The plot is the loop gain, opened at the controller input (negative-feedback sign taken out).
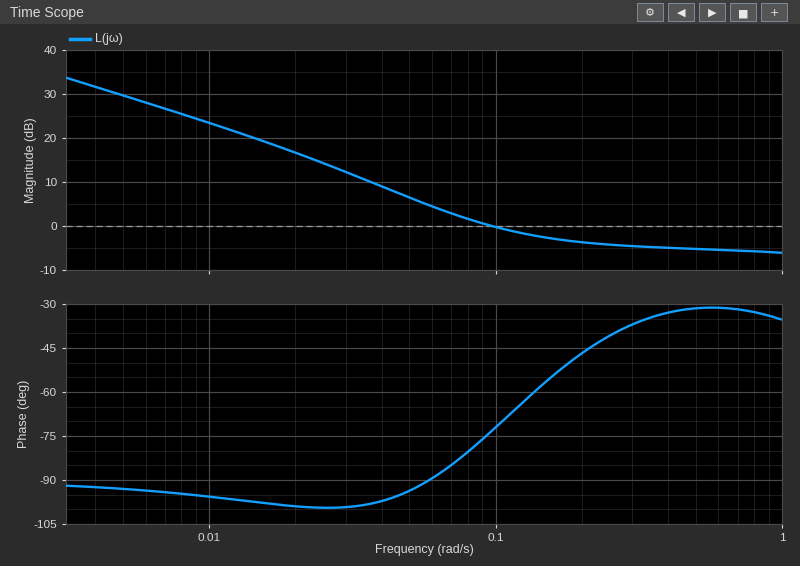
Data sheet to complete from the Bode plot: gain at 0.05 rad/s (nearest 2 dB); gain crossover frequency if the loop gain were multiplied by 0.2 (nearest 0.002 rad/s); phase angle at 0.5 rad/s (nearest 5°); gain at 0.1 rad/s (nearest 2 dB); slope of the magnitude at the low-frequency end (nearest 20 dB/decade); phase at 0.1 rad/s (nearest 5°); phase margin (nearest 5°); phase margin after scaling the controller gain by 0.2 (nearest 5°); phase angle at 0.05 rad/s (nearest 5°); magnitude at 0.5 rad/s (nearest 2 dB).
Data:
6 dB
0.026 rad/s
-30°
0 dB
-20 dB/decade
-70°
105°
80°
-95°
-6 dB
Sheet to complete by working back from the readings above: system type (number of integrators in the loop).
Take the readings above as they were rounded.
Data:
1
